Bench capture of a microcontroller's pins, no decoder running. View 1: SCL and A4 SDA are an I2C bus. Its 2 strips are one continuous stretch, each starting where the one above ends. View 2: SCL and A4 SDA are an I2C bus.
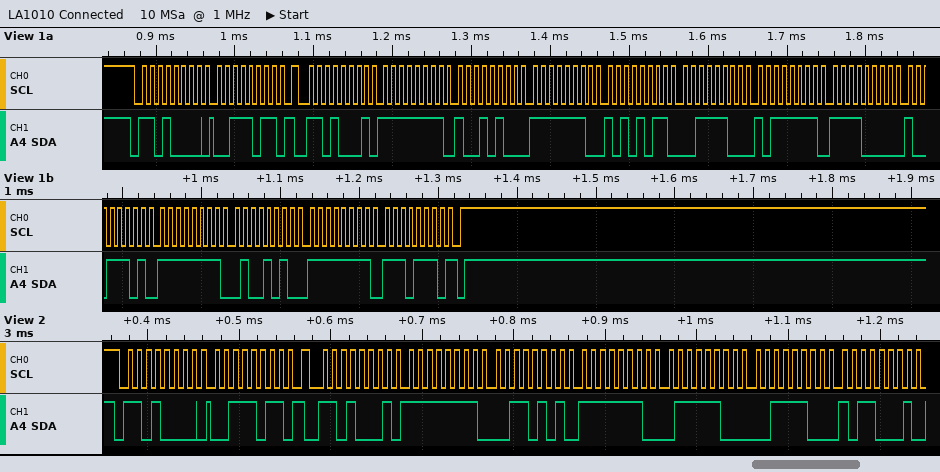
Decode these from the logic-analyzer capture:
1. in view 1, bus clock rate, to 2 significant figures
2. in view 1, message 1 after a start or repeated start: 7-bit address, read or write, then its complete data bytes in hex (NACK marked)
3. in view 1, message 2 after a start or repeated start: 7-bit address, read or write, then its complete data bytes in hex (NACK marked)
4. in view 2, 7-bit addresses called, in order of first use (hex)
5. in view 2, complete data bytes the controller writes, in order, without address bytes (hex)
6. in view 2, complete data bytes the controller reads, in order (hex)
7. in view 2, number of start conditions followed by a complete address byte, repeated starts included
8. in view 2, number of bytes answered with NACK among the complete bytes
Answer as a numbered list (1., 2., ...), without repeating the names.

1. 100 kHz
2. 0x68 write: 3B
3. 0x68 read: FF 94 FE AB 3C BF F0 9D FF 4A FF EE NACK
4. 0x68
5. 3B
6. FF 35 FE 7C 3C B1
7. 2
8. 0
